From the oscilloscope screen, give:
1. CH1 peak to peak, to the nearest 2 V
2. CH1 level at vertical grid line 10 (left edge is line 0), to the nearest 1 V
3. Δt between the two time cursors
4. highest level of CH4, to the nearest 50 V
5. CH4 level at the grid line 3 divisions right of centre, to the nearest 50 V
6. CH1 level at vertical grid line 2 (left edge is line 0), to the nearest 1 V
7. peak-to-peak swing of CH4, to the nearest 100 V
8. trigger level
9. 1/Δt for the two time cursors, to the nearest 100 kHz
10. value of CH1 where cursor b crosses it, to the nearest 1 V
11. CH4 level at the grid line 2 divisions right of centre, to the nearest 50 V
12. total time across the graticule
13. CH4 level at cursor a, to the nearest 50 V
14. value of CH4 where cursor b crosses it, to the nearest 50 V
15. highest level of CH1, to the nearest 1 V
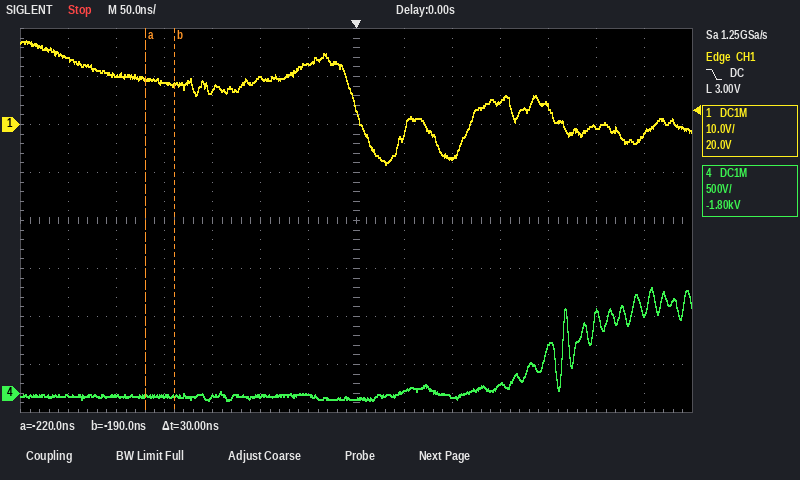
26 V
5 V
30 ns
1.10 kV
100 V
10 V
1.20 kV
3.00 V
33.3 MHz
8 V
-50 V
700 ns
-50 V
-50 V
18 V
